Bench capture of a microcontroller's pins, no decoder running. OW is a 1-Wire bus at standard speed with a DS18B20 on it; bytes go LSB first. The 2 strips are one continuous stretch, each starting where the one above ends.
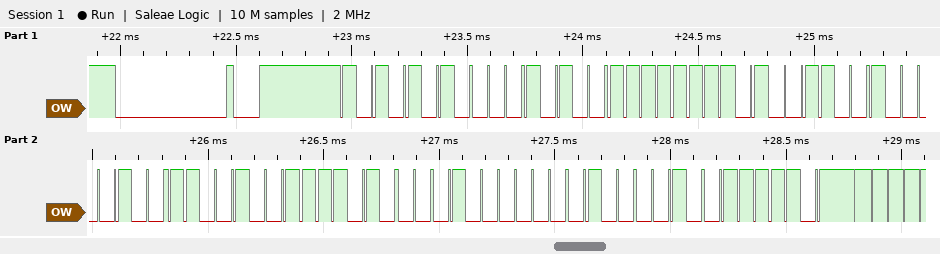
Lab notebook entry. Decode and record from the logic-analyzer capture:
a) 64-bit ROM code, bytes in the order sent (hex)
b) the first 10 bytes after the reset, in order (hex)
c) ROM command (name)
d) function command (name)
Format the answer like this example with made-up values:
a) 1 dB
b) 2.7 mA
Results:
a) 28 FF 32 21 93 17 02 42
b) 55 28 FF 32 21 93 17 02 42 BE
c) Match ROM
d) Read Scratchpad
